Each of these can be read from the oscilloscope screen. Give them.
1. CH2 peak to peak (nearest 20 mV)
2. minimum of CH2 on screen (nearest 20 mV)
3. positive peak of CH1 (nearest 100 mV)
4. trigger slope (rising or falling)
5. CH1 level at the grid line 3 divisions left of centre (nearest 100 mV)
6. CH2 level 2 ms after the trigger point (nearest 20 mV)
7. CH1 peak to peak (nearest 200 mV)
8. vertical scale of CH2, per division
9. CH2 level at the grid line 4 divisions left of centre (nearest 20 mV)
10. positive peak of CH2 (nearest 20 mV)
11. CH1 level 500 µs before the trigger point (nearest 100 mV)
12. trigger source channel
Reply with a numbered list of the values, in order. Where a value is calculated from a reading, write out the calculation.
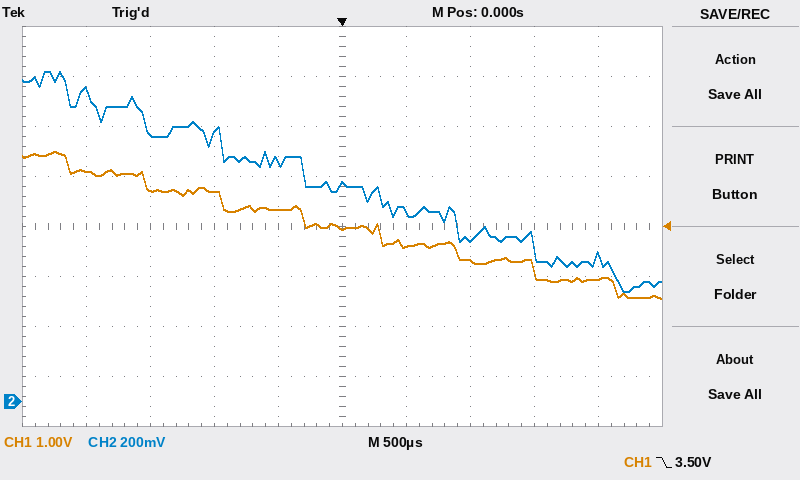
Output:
1. 1.32 V − (440 mV) = 880 mV
2. 440 mV
3. 5.0 V
4. falling
5. 4.2 V
6. 580 mV
7. 3.0 V
8. 200 mV
9. 1.24 V
10. 1.32 V
11. 3.8 V
12. CH1
